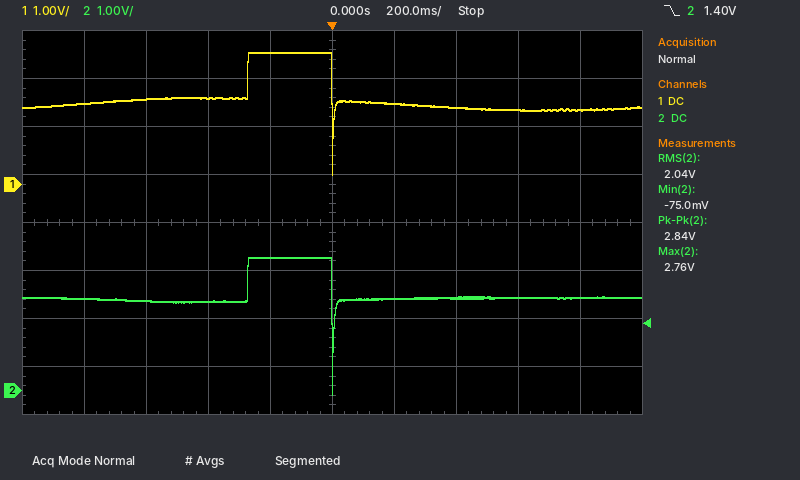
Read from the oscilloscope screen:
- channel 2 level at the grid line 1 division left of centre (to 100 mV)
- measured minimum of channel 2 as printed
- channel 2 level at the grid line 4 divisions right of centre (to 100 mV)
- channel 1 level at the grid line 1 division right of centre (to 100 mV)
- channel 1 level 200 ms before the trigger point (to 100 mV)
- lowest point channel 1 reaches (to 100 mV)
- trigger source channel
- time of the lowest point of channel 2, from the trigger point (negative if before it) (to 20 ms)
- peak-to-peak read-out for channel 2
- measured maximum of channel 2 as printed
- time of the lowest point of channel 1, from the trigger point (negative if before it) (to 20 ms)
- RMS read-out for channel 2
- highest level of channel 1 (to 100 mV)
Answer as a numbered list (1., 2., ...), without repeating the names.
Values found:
1. 2.8 V
2. -75.0 mV
3. 1.9 V
4. 1.7 V
5. 2.7 V
6. 200 mV
7. channel 2
8. 0 ms
9. 2.84 V
10. 2.76 V
11. 0 ms
12. 2.04 V
13. 2.7 V
